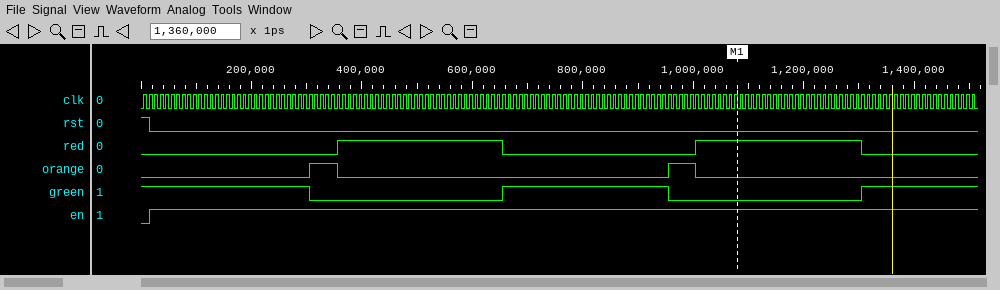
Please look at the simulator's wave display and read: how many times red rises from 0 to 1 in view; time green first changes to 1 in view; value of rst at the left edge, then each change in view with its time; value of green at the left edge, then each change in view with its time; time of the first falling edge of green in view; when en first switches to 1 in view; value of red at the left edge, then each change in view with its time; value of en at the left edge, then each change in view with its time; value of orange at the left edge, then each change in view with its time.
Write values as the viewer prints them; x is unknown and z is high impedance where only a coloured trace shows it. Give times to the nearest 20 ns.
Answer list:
2
660 ns
1, 0 at 20 ns
1, 0 at 300 ns, 1 at 660 ns, 0 at 960 ns, 1 at 1300 ns
300 ns
20 ns
0, 1 at 360 ns, 0 at 660 ns, 1 at 1000 ns, 0 at 1300 ns
0, 1 at 20 ns
0, 1 at 300 ns, 0 at 360 ns, 1 at 960 ns, 0 at 1000 ns
